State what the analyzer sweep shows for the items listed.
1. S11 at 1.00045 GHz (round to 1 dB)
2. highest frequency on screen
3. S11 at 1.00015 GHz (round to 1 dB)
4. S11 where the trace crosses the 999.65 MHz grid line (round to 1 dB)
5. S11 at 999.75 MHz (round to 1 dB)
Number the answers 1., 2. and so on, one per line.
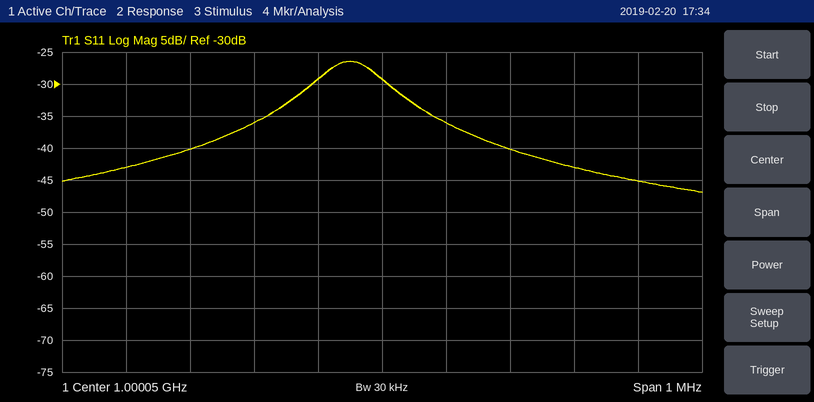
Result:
1. -45 dB
2. 1.00055 GHz
3. -36 dB
4. -43 dB
5. -40 dB
